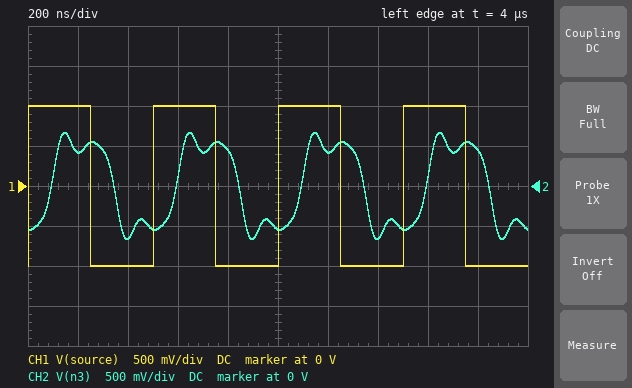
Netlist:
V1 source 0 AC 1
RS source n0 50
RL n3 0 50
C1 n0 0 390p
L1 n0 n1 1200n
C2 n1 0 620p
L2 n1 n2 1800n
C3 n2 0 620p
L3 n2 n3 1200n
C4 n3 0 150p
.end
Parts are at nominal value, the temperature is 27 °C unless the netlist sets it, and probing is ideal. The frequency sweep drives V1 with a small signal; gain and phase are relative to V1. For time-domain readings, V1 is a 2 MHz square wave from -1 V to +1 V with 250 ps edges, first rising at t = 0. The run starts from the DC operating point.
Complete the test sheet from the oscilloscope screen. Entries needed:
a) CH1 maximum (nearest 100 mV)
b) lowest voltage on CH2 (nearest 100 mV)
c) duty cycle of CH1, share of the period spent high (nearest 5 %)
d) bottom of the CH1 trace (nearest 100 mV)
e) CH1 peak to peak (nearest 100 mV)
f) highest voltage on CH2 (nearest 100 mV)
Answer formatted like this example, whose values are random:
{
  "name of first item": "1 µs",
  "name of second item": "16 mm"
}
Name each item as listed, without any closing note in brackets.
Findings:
{
  "CH1 maximum": "1.0 V",
  "lowest voltage on CH2": "-700 mV",
  "duty cycle of CH1, share of the period spent high": "50 %",
  "bottom of the CH1 trace": "-1.0 V",
  "CH1 peak to peak": "2.0 V",
  "highest voltage on CH2": "700 mV"
}
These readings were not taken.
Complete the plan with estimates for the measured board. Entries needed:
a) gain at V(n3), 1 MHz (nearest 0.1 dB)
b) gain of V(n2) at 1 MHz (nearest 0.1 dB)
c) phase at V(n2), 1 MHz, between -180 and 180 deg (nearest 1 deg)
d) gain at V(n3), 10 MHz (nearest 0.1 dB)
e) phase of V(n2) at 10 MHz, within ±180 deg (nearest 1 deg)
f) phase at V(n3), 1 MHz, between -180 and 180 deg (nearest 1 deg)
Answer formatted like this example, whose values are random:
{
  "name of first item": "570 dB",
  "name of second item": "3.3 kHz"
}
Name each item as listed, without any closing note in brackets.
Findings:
{
  "gain at V(n3), 1 MHz": "-6.0 dB",
  "gain of V(n2) at 1 MHz": "-6.0 dB",
  "phase at V(n2), 1 MHz, between -180 and 180 deg": "-23 deg",
  "gain at V(n3), 10 MHz": "-11.8 dB",
  "phase of V(n2) at 10 MHz, within ±180 deg": "36 deg",
  "phase at V(n3), 1 MHz, between -180 and 180 deg": "-31 deg"
}
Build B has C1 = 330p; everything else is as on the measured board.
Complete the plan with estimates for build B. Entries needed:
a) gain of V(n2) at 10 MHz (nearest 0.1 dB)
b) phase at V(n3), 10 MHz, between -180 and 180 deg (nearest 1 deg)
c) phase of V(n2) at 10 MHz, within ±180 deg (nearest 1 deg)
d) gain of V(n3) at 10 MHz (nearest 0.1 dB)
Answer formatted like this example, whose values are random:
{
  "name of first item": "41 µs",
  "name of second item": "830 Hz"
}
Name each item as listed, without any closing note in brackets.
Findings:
{
  "gain of V(n2) at 10 MHz": "-8.3 dB",
  "phase at V(n3), 10 MHz, between -180 and 180 deg": "-33 deg",
  "phase of V(n2) at 10 MHz, within ±180 deg": "46 deg",
  "gain of V(n3) at 10 MHz": "-12.0 dB"
}
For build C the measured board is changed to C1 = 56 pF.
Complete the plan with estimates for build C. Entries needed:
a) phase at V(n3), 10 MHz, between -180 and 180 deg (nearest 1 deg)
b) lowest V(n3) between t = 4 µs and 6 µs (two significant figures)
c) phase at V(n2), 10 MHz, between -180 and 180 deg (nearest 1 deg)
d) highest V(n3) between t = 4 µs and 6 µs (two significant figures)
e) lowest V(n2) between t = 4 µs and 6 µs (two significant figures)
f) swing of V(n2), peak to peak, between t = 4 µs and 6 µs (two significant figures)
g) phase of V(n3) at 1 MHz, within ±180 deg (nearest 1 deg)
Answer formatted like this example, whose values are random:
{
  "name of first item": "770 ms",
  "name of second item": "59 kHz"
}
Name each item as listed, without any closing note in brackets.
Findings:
{
  "phase at V(n3), 10 MHz, between -180 and 180 deg": "-1 deg",
  "lowest V(n3) between t = 4 µs and 6 µs": "-650 mV",
  "phase at V(n2), 10 MHz, between -180 and 180 deg": "78 deg",
  "highest V(n3) between t = 4 µs and 6 µs": "650 mV",
  "lowest V(n2) between t = 4 µs and 6 µs": "-710 mV",
  "swing of V(n2), peak to peak, between t = 4 µs and 6 µs": "1.4 V",
  "phase of V(n3) at 1 MHz, within ±180 deg": "-28 deg"
}
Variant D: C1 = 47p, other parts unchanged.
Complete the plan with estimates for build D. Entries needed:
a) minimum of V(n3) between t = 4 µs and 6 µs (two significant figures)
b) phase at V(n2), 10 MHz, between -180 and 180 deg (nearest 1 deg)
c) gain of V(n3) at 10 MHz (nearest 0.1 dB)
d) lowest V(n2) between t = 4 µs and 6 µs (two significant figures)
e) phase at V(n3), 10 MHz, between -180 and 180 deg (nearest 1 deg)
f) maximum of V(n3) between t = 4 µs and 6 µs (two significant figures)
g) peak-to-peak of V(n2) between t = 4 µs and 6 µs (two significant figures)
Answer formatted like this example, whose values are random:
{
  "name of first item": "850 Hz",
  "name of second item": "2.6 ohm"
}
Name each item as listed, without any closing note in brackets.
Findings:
{
  "minimum of V(n3) between t = 4 µs and 6 µs": "-650 mV",
  "phase at V(n2), 10 MHz, between -180 and 180 deg": "79 deg",
  "gain of V(n3) at 10 MHz": "-15.1 dB",
  "lowest V(n2) between t = 4 µs and 6 µs": "-710 mV",
  "phase at V(n3), 10 MHz, between -180 and 180 deg": "0 deg",
  "maximum of V(n3) between t = 4 µs and 6 µs": "650 mV",
  "peak-to-peak of V(n2) between t = 4 µs and 6 µs": "1.4 V"
}
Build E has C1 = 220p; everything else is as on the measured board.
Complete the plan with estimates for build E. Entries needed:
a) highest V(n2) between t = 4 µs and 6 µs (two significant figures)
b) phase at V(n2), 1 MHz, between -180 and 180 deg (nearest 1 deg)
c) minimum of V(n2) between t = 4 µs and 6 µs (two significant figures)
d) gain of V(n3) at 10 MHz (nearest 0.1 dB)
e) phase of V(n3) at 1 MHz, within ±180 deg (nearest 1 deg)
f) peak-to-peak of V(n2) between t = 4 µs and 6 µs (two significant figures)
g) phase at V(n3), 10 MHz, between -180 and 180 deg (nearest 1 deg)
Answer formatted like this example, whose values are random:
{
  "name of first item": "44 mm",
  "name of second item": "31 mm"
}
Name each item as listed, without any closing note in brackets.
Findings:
{
  "highest V(n2) between t = 4 µs and 6 µs": "730 mV",
  "phase at V(n2), 1 MHz, between -180 and 180 deg": "-21 deg",
  "minimum of V(n2) between t = 4 µs and 6 µs": "-730 mV",
  "gain of V(n3) at 10 MHz": "-13.0 dB",
  "phase of V(n3) at 1 MHz, within ±180 deg": "-30 deg",
  "peak-to-peak of V(n2) between t = 4 µs and 6 µs": "1.5 V",
  "phase at V(n3), 10 MHz, between -180 and 180 deg": "-18 deg"
}
